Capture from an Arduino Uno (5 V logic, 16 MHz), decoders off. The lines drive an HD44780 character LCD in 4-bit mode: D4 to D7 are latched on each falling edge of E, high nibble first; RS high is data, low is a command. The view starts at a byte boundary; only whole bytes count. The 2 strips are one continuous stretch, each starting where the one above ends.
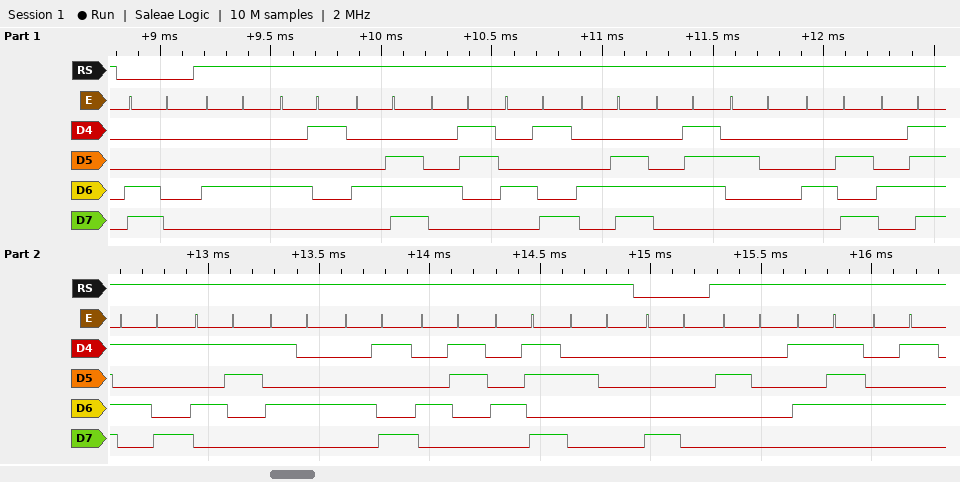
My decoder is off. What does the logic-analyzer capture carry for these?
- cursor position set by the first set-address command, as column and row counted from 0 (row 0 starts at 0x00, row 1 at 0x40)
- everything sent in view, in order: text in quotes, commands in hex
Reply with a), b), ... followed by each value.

a) column 0, row 1
b) 0xC0 "DANCING JOYSTICK " 0x80 " WE"
